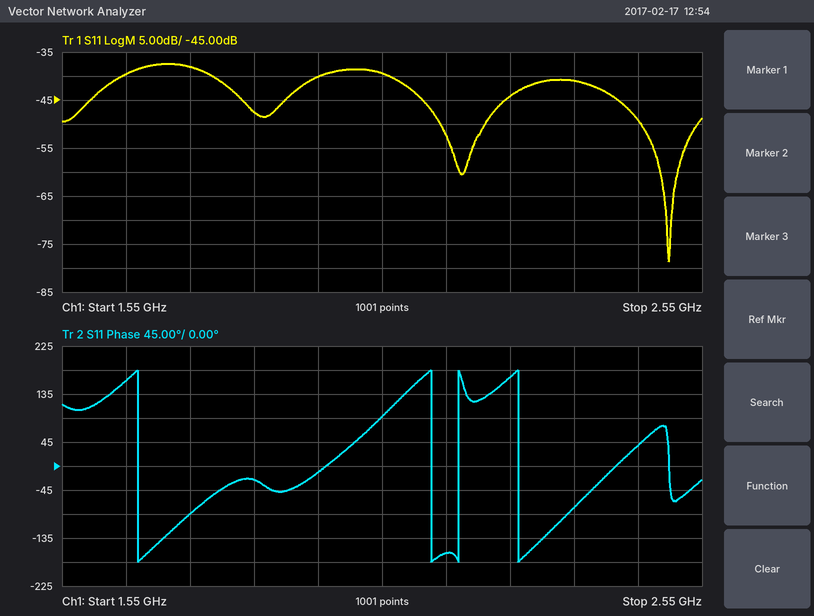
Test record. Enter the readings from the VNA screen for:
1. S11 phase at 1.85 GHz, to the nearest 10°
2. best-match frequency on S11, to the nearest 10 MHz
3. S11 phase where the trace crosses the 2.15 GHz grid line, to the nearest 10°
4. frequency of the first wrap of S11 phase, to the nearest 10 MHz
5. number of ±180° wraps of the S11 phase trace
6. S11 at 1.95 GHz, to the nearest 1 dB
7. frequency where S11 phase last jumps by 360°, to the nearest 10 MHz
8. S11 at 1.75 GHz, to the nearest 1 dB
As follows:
-30°
2.50 GHz
-160°
1.67 GHz
4
-40 dB
2.26 GHz
-38 dB
